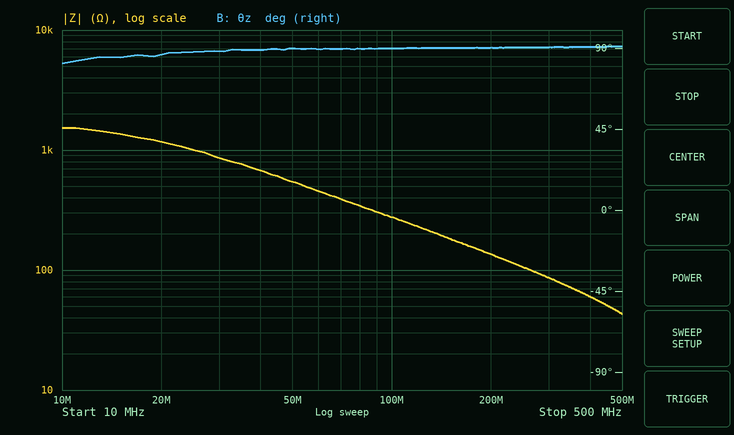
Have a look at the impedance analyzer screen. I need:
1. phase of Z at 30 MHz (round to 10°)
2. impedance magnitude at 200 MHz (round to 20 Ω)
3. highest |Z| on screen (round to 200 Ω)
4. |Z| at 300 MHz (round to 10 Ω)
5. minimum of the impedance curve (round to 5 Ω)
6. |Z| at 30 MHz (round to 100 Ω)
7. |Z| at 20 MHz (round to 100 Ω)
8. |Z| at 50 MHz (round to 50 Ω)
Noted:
90°
140 Ω
1.6 kΩ
90 Ω
45 Ω
900 Ω
1.2 kΩ
550 Ω
